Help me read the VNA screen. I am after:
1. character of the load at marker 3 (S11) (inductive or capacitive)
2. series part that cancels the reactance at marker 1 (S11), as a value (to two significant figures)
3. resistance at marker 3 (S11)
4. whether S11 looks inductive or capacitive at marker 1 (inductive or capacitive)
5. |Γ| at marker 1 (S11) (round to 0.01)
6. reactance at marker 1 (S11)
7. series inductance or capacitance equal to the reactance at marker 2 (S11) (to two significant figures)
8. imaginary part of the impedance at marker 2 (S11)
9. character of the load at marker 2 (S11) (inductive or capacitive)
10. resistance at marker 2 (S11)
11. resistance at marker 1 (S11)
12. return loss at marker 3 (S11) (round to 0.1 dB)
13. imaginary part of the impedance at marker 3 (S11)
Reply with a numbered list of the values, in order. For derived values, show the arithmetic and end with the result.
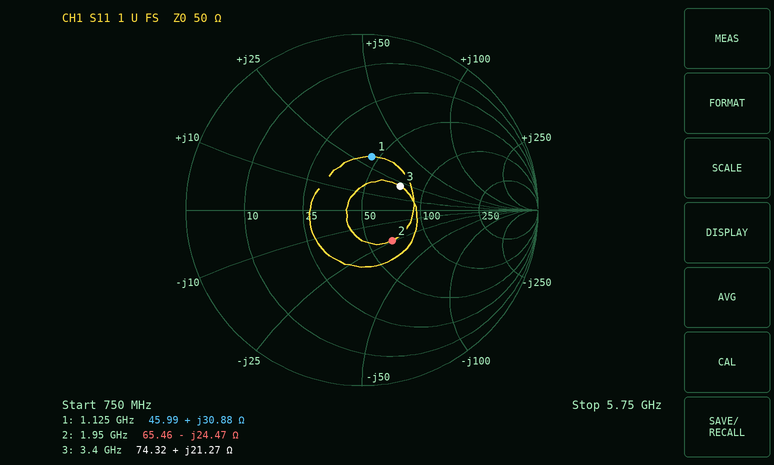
1. inductive
2. C = 1/(2π × 1.125 GHz × 30.88 Ω) ≈ 4.6 pF
3. 74.32 Ω
4. inductive
5. 0.31
6. +30.88 Ω
7. C = 1/(2π × 1.95 GHz × 24.47 Ω) ≈ 3.3 pF
8. -24.47 Ω
9. capacitive
10. 65.46 Ω
11. 45.99 Ω
12. 11.8 dB
13. +21.27 Ω
